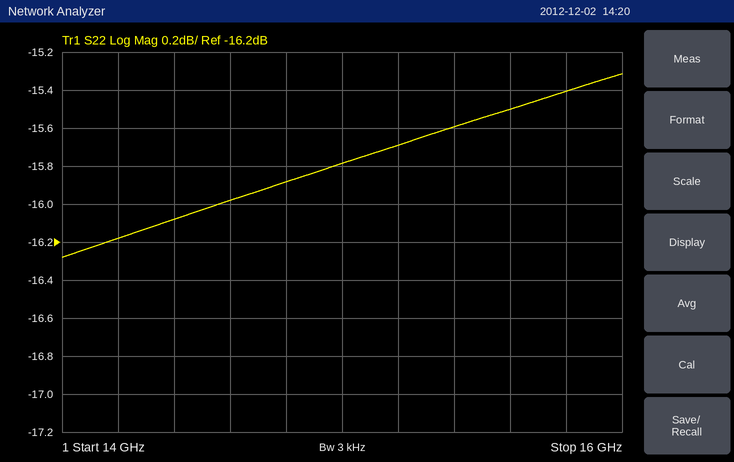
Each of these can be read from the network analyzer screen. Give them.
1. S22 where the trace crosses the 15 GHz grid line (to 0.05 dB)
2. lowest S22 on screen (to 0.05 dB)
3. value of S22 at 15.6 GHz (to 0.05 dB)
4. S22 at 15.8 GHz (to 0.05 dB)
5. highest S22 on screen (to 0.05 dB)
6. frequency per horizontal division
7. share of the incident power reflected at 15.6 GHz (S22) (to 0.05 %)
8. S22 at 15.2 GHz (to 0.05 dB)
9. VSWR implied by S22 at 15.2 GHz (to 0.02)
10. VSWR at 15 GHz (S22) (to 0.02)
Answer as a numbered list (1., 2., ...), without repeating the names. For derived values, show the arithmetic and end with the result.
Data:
1. -15.80 dB
2. -16.30 dB
3. -15.50 dB
4. -15.40 dB
5. -15.30 dB
6. 200 MHz
7. 10^(-15.5/10) ≈ 2.82 %, so 2.80 % to the nearest 0.05 %
8. -15.70 dB
9. |Γ| = 10^(-15.7/20) = 0.1641; VSWR = (1 + 0.1641)/(1 − 0.1641) ≈ 1.39, so 1.40 to the nearest 0.02
10. |Γ| = 10^(-15.8/20) = 0.1622; VSWR = (1 + 0.1622)/(1 − 0.1622) ≈ 1.39, so 1.38 to the nearest 0.02
